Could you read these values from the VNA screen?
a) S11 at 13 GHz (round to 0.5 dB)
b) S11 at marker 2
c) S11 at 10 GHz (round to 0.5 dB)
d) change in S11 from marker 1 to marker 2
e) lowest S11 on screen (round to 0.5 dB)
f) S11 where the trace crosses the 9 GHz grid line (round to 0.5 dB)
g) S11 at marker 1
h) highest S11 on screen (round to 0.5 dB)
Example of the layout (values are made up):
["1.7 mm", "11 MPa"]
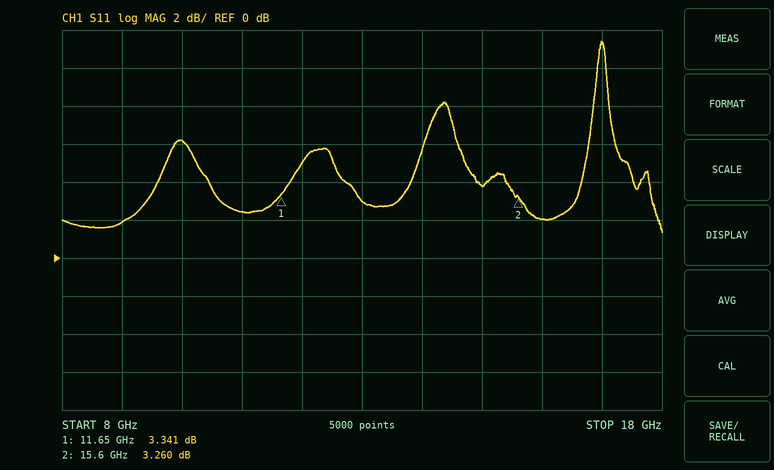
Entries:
["3.0 dB", "3.260 dB", "6.0 dB", "-0.081 dB", "1.5 dB", "2.0 dB", "3.341 dB", "11.5 dB"]
